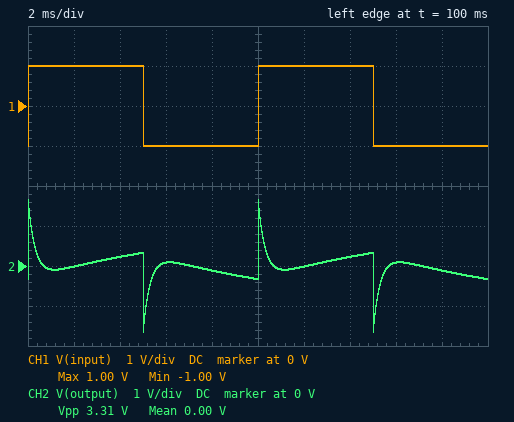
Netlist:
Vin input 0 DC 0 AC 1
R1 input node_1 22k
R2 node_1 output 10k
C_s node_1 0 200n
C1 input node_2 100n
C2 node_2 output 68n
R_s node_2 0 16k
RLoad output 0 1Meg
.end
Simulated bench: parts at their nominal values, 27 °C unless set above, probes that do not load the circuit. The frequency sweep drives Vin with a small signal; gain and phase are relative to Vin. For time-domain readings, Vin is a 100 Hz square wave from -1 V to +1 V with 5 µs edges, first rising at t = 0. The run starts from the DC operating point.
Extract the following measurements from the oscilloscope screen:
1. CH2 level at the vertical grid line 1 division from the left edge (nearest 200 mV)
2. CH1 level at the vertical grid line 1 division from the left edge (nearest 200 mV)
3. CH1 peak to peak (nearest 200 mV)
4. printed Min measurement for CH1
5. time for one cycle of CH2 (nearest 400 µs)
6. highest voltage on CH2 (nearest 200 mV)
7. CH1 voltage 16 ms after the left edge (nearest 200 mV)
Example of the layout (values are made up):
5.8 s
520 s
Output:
0 V
1.0 V
2.0 V
-1.00 V
10.0 ms
1.6 V
-1.0 V
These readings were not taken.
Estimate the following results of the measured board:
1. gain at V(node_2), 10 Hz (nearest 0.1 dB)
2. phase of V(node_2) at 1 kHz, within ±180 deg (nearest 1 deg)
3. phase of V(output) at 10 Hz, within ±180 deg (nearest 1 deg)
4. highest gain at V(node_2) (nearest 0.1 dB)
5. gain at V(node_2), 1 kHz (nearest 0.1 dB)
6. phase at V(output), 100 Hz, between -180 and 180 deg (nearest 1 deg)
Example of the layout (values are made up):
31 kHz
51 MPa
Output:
-16.1 dB
13 deg
-22 deg
0 dB
-0.7 dB
-16 deg
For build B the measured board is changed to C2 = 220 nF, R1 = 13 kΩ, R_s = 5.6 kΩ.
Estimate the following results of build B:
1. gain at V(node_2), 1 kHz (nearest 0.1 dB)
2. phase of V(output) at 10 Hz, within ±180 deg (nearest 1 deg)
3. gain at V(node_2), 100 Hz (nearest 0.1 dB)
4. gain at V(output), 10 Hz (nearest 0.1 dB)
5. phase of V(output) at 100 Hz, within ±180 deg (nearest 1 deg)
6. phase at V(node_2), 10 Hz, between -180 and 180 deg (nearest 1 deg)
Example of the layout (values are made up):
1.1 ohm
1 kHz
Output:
-1.0 dB
-25 deg
-11.7 dB
-1.2 dB
-19 deg
67 deg
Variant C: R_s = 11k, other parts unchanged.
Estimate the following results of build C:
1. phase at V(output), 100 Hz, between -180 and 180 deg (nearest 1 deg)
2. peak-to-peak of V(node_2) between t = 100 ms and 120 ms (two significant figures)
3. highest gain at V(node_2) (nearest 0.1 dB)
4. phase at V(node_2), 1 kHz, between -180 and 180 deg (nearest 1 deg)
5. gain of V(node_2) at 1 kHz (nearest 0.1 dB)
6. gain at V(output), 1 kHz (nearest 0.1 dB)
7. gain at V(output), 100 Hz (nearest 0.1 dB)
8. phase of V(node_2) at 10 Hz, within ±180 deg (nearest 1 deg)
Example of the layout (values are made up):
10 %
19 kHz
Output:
-53 deg
3.7 V
0 dB
15 deg
-0.8 dB
-1.2 dB
-25.1 dB
75 deg
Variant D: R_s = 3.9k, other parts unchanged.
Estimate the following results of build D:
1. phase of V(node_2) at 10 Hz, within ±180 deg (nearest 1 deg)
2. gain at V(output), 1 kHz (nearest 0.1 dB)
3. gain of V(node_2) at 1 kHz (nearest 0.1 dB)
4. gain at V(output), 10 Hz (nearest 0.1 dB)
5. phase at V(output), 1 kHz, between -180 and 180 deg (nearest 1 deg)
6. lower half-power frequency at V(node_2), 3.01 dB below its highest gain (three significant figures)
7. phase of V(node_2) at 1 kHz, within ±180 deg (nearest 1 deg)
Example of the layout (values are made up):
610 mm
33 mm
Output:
79 deg
-2.0 dB
-1.5 dB
-0.9 dB
41 deg
623 Hz
28 deg
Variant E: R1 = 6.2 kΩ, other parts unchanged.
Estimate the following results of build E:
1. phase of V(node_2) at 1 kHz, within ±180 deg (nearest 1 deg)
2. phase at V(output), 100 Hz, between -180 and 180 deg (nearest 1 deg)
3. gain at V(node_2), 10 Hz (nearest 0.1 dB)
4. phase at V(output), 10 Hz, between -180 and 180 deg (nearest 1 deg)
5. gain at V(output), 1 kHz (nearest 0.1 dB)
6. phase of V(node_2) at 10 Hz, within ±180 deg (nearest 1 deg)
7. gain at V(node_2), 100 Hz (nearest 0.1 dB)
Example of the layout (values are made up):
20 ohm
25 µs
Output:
13 deg
-38 deg
-15.7 dB
-8 deg
-1.4 dB
77 deg
-3.9 dB
